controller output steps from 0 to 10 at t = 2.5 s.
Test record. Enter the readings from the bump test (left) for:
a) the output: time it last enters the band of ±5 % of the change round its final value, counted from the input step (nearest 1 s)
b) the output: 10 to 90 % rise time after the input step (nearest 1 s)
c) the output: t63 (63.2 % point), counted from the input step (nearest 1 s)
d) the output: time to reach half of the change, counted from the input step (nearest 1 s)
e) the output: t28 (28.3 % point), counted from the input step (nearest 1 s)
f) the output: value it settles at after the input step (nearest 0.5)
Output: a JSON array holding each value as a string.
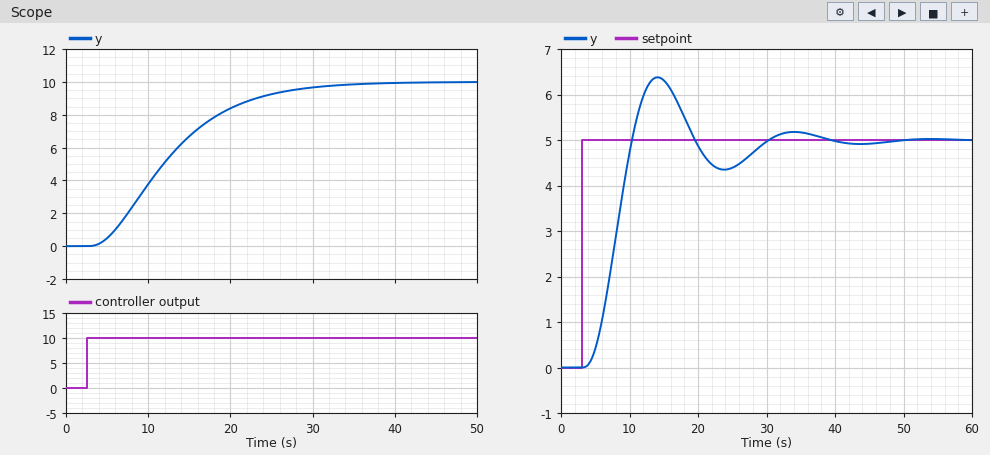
["25 s", "17 s", "12 s", "9 s", "6 s", "10.0"]
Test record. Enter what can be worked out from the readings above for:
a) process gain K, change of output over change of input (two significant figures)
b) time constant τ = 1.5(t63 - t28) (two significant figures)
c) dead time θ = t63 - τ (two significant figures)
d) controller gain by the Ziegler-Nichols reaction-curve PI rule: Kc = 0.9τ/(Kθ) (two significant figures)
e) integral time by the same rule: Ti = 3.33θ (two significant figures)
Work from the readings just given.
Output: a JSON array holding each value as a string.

["1.0", "9.0 s", "3.0 s", "2.7", "10.0 s"]
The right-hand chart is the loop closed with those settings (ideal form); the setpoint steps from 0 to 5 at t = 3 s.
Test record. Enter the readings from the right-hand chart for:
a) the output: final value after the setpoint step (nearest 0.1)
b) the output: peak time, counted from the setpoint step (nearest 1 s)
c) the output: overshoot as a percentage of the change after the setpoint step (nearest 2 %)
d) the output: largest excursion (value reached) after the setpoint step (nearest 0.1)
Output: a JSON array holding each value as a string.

["5.0", "11 s", "28 %", "6.4"]
